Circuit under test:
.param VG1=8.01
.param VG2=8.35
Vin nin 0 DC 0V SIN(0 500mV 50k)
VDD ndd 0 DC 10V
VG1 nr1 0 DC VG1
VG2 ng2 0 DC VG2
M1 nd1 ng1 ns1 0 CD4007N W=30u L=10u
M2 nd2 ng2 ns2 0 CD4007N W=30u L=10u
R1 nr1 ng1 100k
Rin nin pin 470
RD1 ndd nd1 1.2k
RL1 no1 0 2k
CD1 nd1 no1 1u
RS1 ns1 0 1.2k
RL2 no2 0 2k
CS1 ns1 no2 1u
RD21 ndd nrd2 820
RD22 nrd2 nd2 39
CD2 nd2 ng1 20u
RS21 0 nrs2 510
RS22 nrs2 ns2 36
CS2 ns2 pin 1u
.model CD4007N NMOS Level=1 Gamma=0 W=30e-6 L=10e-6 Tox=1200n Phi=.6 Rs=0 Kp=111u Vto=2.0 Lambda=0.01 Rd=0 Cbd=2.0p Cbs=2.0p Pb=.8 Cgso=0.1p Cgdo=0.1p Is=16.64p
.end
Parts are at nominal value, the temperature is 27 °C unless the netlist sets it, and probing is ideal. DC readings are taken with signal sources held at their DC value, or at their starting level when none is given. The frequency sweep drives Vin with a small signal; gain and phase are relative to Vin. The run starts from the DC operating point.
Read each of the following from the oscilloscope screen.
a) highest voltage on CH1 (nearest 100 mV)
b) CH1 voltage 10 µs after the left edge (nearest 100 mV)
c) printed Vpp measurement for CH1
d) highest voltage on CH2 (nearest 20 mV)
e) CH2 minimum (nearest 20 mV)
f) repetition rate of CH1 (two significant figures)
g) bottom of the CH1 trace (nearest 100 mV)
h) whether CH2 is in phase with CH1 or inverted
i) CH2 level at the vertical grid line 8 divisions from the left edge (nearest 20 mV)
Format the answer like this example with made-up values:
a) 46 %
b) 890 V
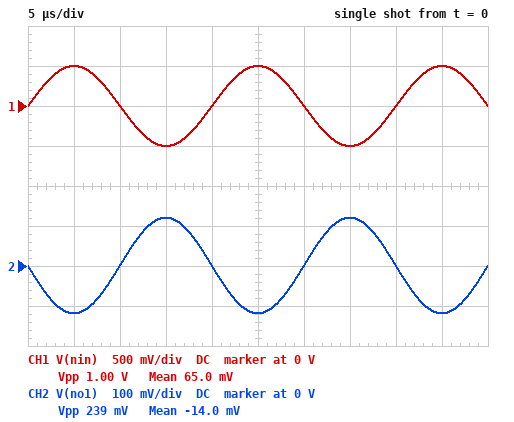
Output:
a) 500 mV
b) 0 V
c) 1.00 V
d) 120 mV
e) -120 mV
f) 50 kHz
g) -500 mV
h) inverted
i) 0 V
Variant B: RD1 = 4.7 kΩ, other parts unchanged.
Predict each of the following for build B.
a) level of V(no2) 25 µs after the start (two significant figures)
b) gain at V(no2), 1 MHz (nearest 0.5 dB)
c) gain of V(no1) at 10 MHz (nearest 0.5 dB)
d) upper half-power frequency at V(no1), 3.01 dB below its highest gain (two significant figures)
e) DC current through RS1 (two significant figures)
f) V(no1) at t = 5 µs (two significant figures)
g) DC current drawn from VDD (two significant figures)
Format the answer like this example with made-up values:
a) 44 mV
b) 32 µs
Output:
a) 21 mV
b) -27.0 dB
c) -21.5 dB
d) 170 MHz
e) 1.5 mA
f) -39 mV
g) 5.0 mA
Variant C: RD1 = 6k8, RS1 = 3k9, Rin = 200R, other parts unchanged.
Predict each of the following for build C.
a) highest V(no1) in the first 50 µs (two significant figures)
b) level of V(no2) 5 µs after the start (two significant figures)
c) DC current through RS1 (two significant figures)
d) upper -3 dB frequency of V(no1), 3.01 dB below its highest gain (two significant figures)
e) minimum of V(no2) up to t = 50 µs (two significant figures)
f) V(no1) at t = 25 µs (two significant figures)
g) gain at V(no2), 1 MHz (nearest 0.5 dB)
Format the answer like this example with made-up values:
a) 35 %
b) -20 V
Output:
a) 87 mV
b) 54 mV
c) 830 µA
d) 200 MHz
e) -74 mV
f) -63 mV
g) -18.0 dB
